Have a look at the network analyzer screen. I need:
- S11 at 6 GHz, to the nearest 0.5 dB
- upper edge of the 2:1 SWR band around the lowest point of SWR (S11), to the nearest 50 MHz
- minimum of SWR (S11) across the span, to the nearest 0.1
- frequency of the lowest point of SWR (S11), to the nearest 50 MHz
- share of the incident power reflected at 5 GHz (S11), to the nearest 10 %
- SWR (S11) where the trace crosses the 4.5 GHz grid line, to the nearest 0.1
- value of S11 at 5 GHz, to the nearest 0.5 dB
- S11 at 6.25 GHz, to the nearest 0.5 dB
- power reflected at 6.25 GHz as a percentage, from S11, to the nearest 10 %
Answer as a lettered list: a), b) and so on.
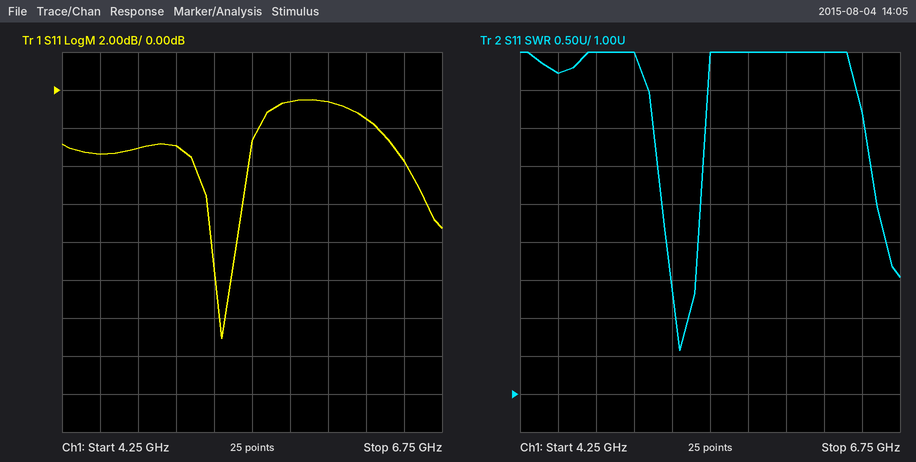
a) -0.5 dB
b) 5.35 GHz
c) 1.6
d) 5.30 GHz
e) 50 %
f) 5.2
g) -3.0 dB
h) -1.5 dB
i) 70 %
